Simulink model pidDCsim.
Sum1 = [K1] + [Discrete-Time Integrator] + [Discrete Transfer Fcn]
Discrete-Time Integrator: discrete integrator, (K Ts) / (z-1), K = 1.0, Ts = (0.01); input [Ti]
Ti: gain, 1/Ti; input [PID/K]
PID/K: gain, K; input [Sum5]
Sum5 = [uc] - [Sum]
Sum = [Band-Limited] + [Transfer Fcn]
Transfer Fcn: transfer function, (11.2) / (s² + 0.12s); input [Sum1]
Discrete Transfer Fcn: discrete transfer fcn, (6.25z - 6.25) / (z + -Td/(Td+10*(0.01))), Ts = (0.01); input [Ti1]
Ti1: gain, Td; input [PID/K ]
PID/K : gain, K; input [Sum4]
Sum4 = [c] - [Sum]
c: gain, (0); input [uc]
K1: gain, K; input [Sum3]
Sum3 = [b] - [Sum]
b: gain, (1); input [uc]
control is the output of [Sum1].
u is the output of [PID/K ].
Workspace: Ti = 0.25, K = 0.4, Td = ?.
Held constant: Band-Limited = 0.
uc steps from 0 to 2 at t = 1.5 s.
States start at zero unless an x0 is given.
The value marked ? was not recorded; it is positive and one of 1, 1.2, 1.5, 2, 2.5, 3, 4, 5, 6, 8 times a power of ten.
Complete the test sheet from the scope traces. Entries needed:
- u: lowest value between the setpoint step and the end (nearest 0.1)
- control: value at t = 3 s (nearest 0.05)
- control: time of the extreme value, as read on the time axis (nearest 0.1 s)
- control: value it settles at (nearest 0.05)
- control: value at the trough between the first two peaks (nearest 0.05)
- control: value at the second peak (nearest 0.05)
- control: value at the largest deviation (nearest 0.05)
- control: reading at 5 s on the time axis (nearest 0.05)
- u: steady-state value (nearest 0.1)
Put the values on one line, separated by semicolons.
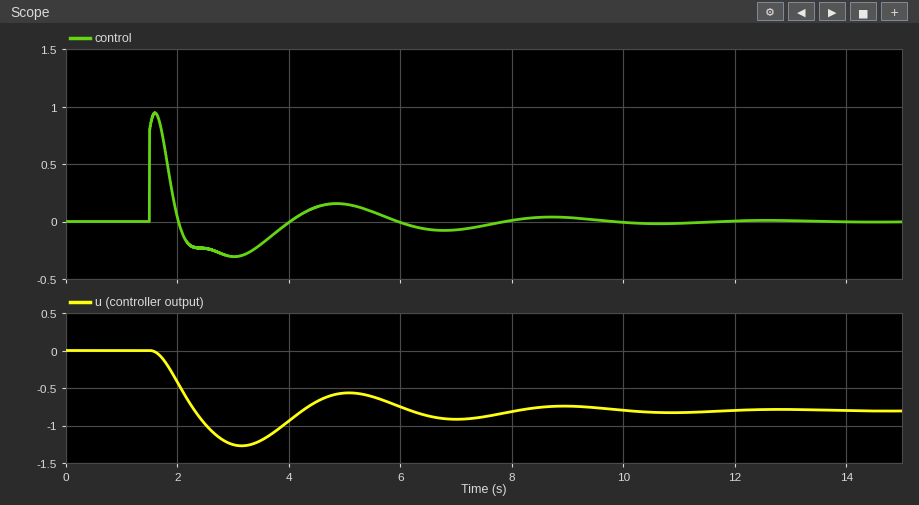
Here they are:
-1.3; -0.30; 1.6 s; 0.00; -0.30; 0.15; 0.95; 0.15; -0.8
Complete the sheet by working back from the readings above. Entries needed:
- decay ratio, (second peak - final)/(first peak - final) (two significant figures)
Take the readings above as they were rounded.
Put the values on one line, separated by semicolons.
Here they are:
0.16
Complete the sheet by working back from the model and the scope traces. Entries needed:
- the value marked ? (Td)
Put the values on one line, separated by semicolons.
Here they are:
1.5
